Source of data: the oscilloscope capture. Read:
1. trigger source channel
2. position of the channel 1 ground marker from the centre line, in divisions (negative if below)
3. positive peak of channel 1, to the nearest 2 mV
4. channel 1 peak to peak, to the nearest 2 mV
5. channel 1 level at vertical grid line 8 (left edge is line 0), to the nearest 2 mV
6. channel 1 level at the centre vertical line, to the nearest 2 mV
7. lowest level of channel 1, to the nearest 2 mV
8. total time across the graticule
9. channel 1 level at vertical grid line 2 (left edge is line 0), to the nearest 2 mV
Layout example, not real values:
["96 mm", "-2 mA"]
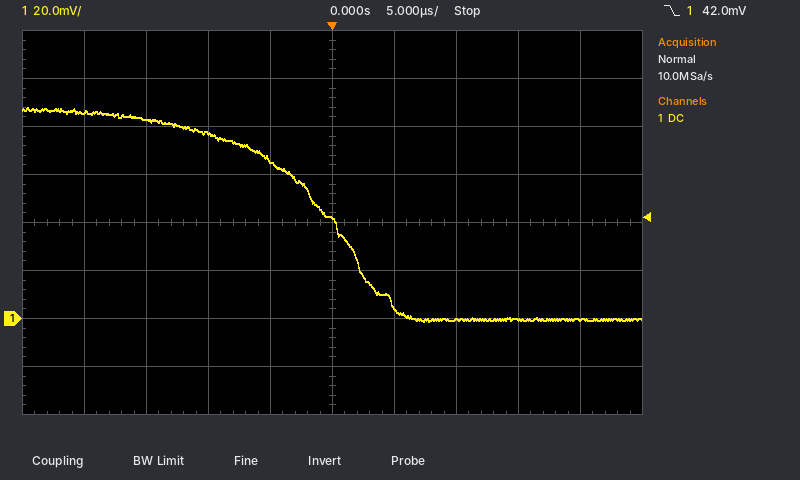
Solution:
["channel 1", "-2.0 div", "88 mV", "90 mV", "0 mV", "42 mV", "-2 mV", "50 µs", "82 mV"]
